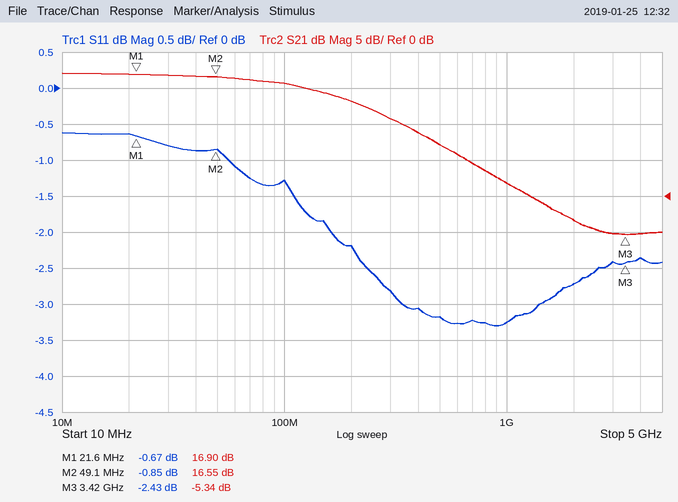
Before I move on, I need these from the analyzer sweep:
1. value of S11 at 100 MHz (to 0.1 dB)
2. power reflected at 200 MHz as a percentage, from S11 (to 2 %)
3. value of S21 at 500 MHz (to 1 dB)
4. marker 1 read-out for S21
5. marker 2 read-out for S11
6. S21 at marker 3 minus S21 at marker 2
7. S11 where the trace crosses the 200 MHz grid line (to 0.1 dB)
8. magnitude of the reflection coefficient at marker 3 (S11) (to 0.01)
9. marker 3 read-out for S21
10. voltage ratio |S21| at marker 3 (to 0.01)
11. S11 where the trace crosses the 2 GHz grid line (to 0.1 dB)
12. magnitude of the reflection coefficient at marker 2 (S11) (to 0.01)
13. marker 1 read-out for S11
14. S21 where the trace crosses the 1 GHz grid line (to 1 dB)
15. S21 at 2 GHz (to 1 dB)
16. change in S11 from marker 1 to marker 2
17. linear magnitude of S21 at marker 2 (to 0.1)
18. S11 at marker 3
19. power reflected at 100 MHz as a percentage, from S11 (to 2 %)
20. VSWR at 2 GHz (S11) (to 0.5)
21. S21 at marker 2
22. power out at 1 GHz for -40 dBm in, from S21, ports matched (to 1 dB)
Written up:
-1.3 dB
60 %
7 dB
16.90 dB
-0.85 dB
-21.89 dB
-2.2 dB
0.76
-5.34 dB
0.54
-2.7 dB
0.91
-0.67 dB
2 dB
-3 dB
-0.18 dB
6.7
-2.43 dB
74 %
6.5
16.55 dB
-38 dBm
